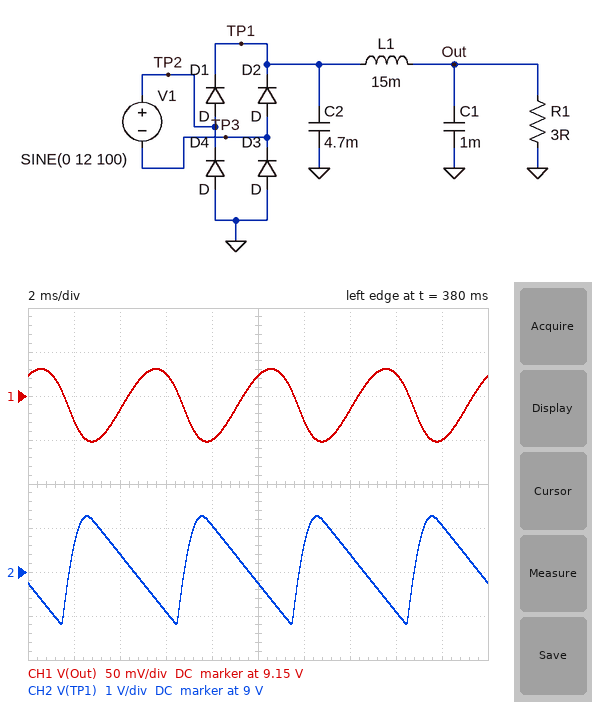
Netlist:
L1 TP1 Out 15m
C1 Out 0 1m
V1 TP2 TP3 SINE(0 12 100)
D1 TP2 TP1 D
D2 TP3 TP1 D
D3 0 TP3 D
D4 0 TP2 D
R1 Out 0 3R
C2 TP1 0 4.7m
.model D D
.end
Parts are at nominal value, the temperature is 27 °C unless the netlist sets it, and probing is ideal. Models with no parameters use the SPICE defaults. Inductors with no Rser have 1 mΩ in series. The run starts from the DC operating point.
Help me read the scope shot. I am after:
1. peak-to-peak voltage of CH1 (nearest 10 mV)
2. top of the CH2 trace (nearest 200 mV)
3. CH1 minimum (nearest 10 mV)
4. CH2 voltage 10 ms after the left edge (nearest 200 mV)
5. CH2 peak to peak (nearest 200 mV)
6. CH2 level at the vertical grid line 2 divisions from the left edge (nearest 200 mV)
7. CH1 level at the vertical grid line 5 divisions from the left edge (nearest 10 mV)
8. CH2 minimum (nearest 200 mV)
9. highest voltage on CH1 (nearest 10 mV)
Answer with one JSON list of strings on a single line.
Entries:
["80 mV", "10.2 V", "9.10 V", "8.8 V", "2.4 V", "9.4 V", "9.17 V", "7.8 V", "9.18 V"]
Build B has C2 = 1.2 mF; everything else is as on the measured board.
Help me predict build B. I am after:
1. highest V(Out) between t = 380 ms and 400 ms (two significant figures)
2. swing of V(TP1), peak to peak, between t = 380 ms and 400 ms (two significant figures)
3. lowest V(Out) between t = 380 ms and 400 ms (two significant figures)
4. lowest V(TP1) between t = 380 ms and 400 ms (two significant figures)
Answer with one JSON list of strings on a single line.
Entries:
["7.7 V", "6.4 V", "7.4 V", "3.9 V"]
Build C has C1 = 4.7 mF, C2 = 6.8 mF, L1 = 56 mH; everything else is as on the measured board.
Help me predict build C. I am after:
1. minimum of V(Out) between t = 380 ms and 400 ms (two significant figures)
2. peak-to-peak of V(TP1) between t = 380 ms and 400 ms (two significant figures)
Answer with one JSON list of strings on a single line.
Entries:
["9.4 V", "1.8 V"]
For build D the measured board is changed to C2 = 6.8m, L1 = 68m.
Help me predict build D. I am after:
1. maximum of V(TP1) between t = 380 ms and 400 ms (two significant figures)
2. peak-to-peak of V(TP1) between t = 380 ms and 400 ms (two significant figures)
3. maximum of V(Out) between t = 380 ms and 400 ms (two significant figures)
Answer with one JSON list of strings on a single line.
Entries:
["10 V", "1.8 V", "9.4 V"]
